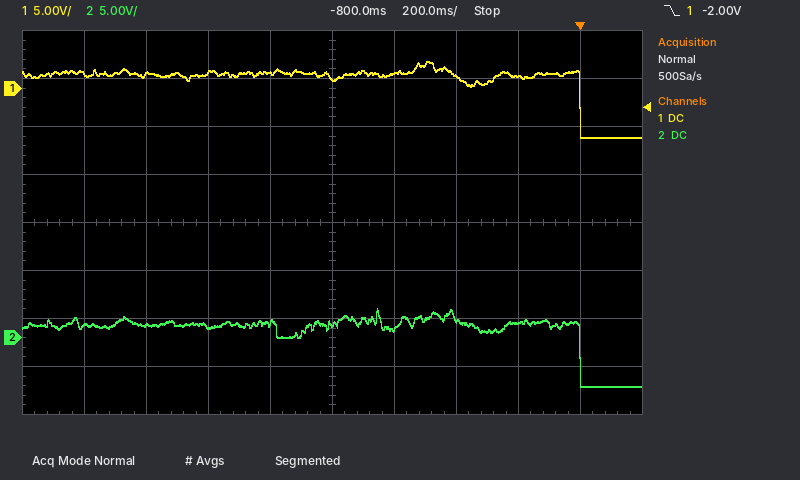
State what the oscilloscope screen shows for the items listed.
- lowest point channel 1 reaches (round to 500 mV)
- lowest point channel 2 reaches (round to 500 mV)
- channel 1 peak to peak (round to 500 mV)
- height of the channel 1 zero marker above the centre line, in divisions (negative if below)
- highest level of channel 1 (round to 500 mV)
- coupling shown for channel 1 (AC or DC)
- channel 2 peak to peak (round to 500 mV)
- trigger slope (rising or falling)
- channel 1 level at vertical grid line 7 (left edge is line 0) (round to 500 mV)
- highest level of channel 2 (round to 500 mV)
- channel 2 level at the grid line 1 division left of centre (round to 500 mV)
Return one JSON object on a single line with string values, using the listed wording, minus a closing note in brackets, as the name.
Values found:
{"lowest point channel 1 reaches": "-5.0 V", "lowest point channel 2 reaches": "-5.0 V", "channel 1 peak to peak": "8.0 V", "height of the channel 1 zero marker above the centre line, in divisions": "+2.8 div", "highest level of channel 1": "3.0 V", "coupling shown for channel 1": "DC", "channel 2 peak to peak": "8.0 V", "trigger slope": "falling", "channel 1 level at vertical grid line 7 (left edge is line 0)": "1.5 V", "highest level of channel 2": "3.0 V", "channel 2 level at the grid line 1 division left of centre": "1.5 V"}
